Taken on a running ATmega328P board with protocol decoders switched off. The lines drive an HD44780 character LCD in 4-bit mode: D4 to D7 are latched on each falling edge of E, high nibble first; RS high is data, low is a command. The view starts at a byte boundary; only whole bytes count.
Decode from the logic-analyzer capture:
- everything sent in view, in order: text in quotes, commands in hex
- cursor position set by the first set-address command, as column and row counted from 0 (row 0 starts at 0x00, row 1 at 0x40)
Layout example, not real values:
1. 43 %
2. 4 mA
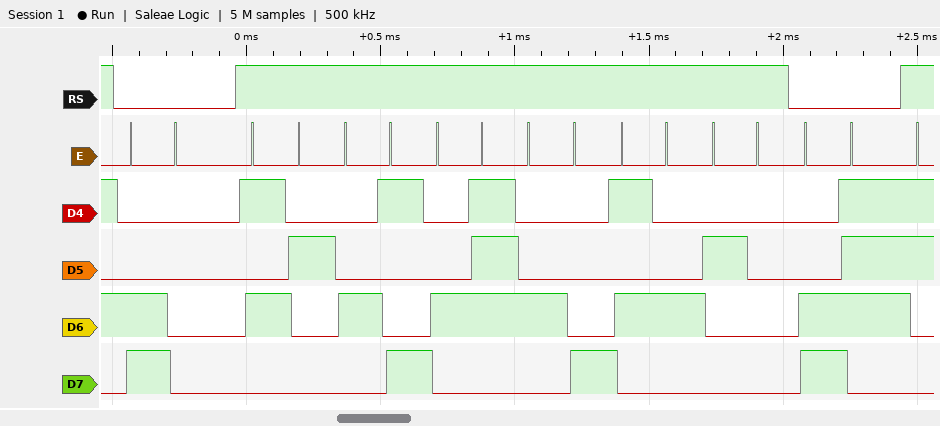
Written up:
1. 0xC0 "RIGHT " 0xC7
2. column 0, row 1
